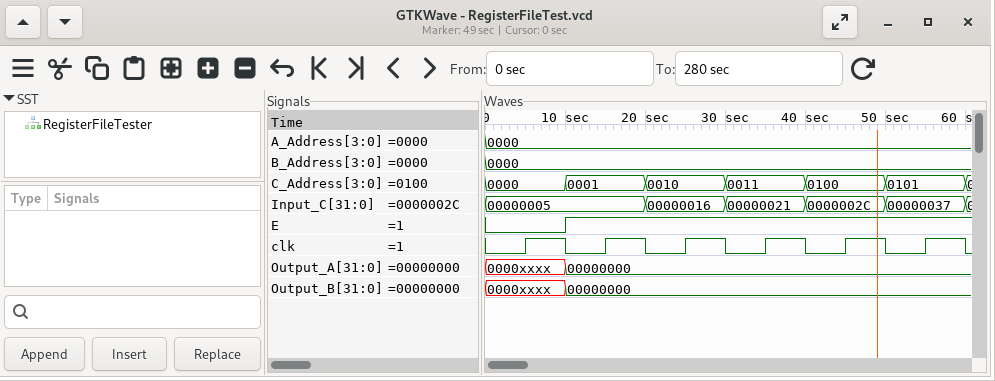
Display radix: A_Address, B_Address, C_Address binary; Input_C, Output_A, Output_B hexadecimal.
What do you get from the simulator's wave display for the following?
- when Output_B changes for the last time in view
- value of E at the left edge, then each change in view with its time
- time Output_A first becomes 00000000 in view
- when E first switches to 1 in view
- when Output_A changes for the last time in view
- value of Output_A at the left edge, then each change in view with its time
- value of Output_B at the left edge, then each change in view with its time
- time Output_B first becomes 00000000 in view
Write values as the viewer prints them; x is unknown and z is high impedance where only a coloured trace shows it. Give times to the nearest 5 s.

10 s
0, 1 at 10 s
10 s
10 s
10 s
0000xxxx, 00000000 at 10 s
0000xxxx, 00000000 at 10 s
10 s
